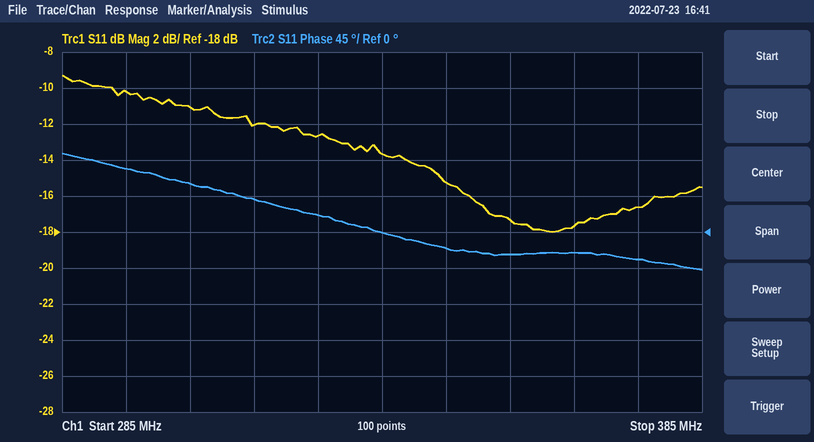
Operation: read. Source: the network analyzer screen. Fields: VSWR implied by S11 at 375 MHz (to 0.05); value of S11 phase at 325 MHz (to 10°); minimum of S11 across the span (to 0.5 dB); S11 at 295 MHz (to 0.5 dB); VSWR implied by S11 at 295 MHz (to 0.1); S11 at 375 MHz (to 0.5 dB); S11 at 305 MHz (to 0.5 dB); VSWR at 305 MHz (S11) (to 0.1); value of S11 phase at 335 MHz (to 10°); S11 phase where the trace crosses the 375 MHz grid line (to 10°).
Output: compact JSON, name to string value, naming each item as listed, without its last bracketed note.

{"VSWR implied by S11 at 375 MHz": "1.35", "value of S11 phase at 325 MHz": "20°", "minimum of S11 across the span": "-18.0 dB", "S11 at 295 MHz": "-10.0 dB", "VSWR implied by S11 at 295 MHz": "1.9", "S11 at 375 MHz": "-16.5 dB", "S11 at 305 MHz": "-11.0 dB", "VSWR at 305 MHz (S11)": "1.8", "value of S11 phase at 335 MHz": "0°", "S11 phase where the trace crosses the 375 MHz grid line": "-30°"}
